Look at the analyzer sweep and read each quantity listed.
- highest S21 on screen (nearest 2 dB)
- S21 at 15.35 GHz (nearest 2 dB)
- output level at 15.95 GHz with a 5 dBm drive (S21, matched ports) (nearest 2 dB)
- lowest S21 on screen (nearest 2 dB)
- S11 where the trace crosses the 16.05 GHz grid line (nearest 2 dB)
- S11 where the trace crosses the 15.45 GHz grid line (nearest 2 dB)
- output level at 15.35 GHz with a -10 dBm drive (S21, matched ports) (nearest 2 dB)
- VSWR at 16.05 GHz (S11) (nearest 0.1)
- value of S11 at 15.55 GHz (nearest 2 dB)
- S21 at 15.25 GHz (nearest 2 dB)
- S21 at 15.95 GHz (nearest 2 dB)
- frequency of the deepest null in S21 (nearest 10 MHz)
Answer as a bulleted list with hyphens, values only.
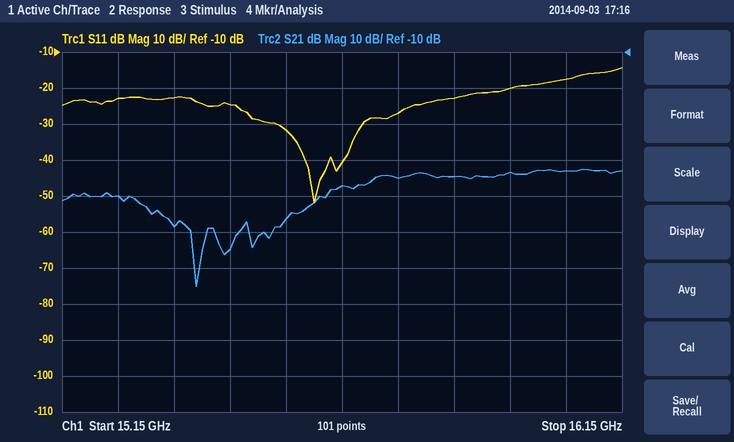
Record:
- -42 dB
- -58 dB
- -38 dBm
- -76 dB
- -18 dB
- -24 dB
- -68 dBm
- 1.3
- -32 dB
- -50 dB
- -44 dB
- 15.39 GHz
